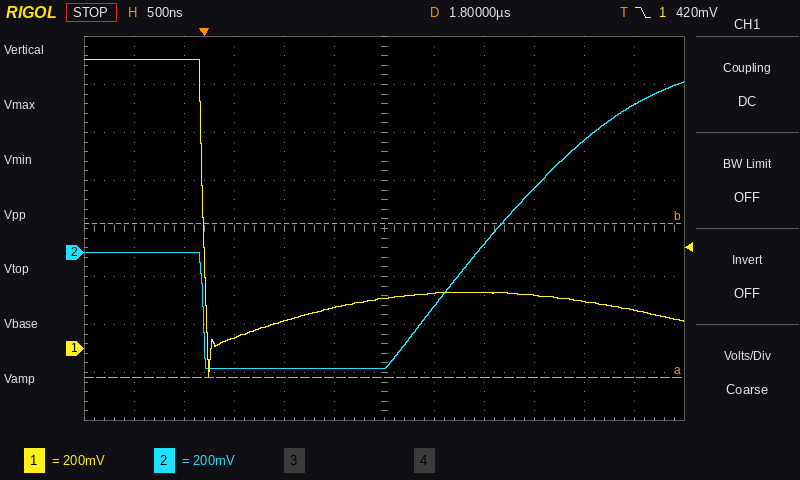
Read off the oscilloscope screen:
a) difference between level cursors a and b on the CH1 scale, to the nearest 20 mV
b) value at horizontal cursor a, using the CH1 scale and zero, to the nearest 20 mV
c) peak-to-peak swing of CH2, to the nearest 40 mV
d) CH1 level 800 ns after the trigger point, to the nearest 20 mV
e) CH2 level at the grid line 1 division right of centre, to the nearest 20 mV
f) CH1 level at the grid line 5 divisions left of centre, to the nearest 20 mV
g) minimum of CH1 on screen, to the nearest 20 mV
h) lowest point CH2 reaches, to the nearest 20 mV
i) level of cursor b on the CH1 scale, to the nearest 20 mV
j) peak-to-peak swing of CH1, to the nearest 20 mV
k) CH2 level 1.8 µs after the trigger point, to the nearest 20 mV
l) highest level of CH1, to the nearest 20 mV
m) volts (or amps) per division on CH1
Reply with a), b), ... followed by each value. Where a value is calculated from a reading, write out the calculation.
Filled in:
a) 640 mV
b) -120 mV
c) 1.20 V
d) 120 mV
e) -220 mV
f) 1.20 V
g) -120 mV
h) -480 mV
i) 520 mV
j) 1.20 V − (-120 mV) = 1.32 V
k) -480 mV
l) 1.20 V
m) 200 mV
